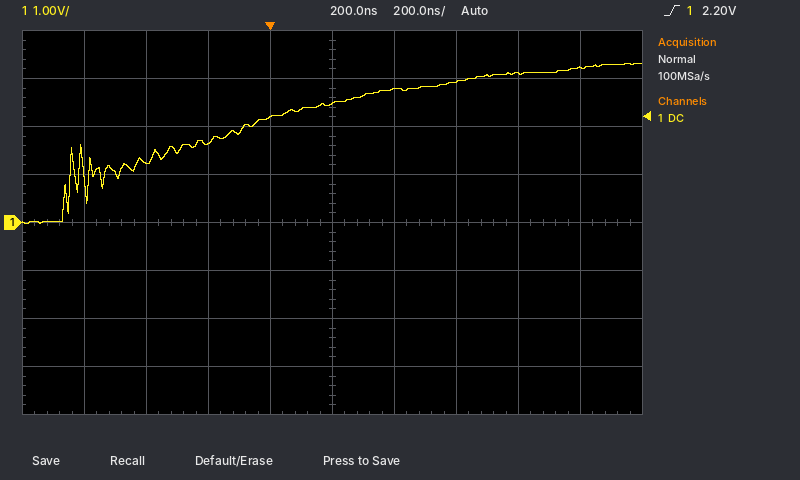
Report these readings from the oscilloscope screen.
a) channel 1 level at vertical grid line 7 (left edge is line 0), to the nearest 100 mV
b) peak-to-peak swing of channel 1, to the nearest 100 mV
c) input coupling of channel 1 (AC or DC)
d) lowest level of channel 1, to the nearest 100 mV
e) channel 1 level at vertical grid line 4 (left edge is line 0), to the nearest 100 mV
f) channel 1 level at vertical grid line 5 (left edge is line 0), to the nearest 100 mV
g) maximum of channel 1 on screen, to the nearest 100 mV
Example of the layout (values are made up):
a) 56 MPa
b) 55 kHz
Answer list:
a) 2.9 V
b) 3.3 V
c) DC
d) 0.0 V
e) 2.2 V
f) 2.5 V
g) 3.3 V
